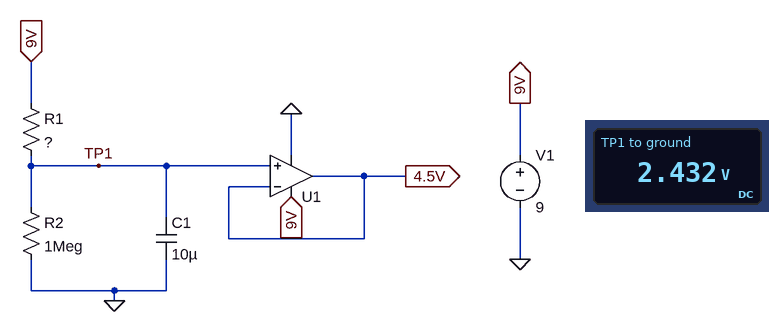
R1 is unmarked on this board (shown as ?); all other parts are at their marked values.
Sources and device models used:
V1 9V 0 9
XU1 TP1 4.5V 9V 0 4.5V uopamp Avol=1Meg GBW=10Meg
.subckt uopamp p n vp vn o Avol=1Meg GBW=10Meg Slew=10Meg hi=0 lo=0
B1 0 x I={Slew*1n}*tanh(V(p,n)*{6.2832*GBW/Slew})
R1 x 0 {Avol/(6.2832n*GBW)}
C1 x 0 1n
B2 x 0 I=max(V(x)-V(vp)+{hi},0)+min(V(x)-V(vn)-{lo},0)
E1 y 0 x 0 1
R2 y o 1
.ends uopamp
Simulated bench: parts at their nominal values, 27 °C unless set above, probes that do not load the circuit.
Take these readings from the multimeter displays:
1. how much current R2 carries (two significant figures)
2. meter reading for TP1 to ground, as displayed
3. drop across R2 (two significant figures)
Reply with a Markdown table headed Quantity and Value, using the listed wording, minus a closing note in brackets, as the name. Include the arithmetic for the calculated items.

| Quantity | Value |
|---|---|
| how much current R2 carries | (2.432 V) / 1 MΩ = 2.4 µA |
| meter reading for TP1 to ground, as displayed | 2.432 V |
| drop across R2 | 2.432 V = 2.4 V |
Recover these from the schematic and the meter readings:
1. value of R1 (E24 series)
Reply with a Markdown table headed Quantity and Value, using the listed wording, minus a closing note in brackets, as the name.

| Quantity | Value |
|---|---|
| value of R1 | 2.7 MΩ |
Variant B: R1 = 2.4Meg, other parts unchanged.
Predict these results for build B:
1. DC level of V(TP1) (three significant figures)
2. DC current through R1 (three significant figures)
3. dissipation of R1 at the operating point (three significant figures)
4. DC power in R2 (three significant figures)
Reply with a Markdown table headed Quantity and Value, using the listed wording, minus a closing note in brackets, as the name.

| Quantity | Value |
|---|---|
| DC level of V(TP1) | 2.65 V |
| DC current through R1 | 2.65 µA |
| dissipation of R1 at the operating point | 16.8 µW |
| DC power in R2 | 7.01 µW |
